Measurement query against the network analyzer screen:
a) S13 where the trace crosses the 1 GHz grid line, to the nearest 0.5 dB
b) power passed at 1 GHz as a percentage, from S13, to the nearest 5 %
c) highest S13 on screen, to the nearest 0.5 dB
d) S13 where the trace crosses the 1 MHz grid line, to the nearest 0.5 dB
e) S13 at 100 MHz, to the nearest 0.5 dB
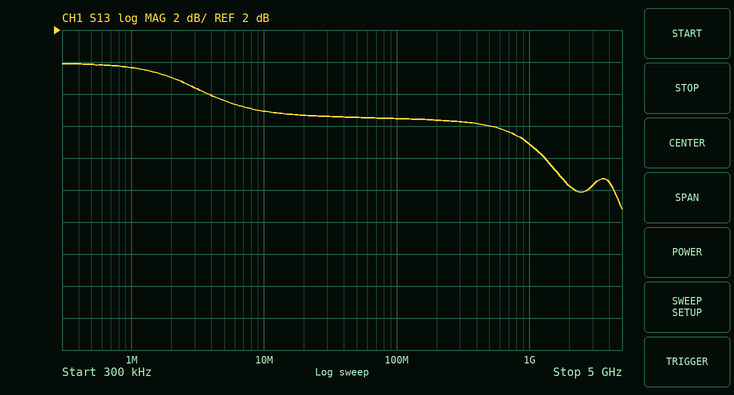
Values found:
-5.0 dB
30 %
0.0 dB
-0.5 dB
-3.5 dB
